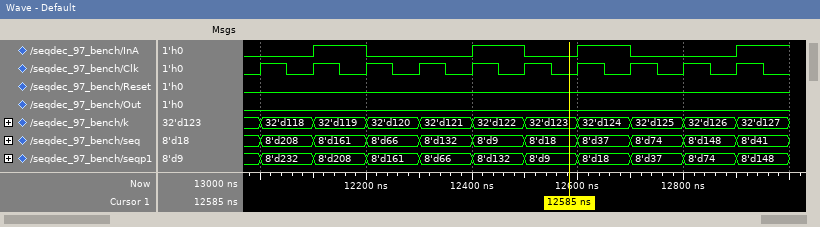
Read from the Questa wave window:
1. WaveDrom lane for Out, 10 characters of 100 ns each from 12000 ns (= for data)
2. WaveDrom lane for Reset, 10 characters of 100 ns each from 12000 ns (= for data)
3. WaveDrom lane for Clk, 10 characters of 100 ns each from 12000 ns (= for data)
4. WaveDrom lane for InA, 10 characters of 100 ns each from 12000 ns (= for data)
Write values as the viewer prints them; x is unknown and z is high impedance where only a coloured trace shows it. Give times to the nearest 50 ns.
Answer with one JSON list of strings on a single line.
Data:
["{name: 'Out', wave: '0.........'}", "{name: 'Reset', wave: '0.........'}", "{name: 'Clk', wave: 'p.........'}", "{name: 'InA', wave: '010.1010.1'}"]
